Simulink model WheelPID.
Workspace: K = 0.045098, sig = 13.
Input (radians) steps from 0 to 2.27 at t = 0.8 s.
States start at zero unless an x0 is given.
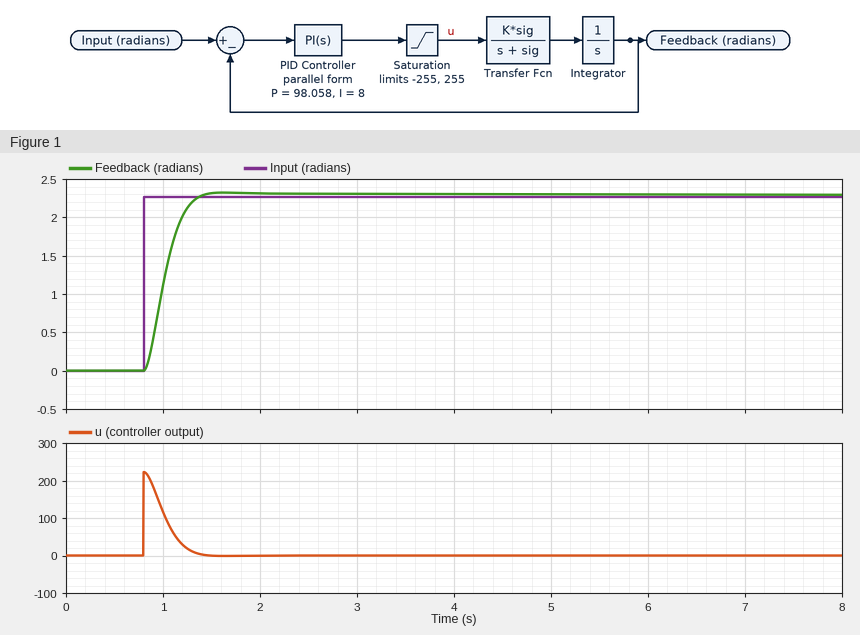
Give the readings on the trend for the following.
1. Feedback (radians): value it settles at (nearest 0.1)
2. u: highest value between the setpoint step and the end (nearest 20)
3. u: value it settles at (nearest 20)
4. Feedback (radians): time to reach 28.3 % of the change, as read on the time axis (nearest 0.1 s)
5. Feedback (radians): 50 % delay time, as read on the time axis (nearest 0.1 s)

2.3
220
0
0.9 s
1.0 s
